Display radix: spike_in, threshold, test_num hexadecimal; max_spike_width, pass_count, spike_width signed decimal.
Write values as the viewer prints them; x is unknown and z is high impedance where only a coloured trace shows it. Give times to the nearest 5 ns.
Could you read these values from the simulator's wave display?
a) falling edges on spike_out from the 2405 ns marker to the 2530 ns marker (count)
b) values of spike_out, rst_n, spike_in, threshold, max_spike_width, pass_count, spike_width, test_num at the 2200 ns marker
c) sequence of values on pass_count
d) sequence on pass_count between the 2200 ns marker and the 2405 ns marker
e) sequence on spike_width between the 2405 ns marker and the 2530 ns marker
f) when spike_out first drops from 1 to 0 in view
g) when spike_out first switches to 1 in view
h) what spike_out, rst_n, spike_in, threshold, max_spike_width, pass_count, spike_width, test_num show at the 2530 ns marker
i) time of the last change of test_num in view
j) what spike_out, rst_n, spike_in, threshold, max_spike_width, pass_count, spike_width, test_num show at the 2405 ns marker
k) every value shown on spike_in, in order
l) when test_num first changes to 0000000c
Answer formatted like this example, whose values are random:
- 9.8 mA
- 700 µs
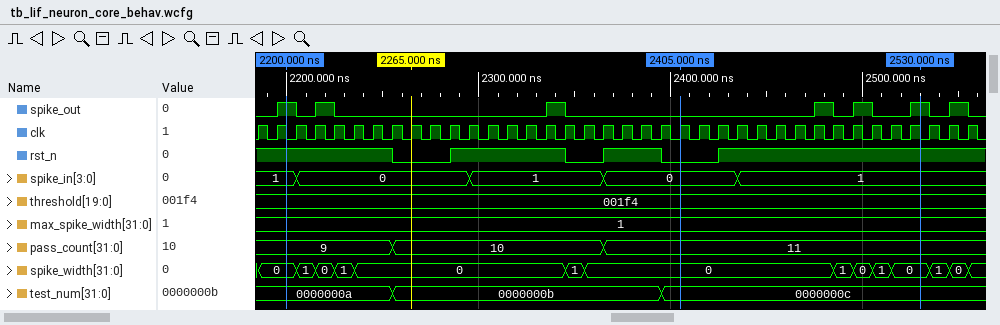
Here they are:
- 2
- spike_out=1, rst_n=1, spike_in=1, threshold=001f4, max_spike_width=1, pass_count=9, spike_width=0, test_num=0000000a
- 9, 10, 11
- 9, 10, 11
- 0, 1, 0, 1, 0
- 2205 ns
- 2195 ns
- spike_out=1, rst_n=1, spike_in=1, threshold=001f4, max_spike_width=1, pass_count=11, spike_width=0, test_num=0000000c
- 2395 ns
- spike_out=0, rst_n=0, spike_in=0, threshold=001f4, max_spike_width=1, pass_count=11, spike_width=0, test_num=0000000c
- 1, 0, 1, 0, 1
- 2395 ns
